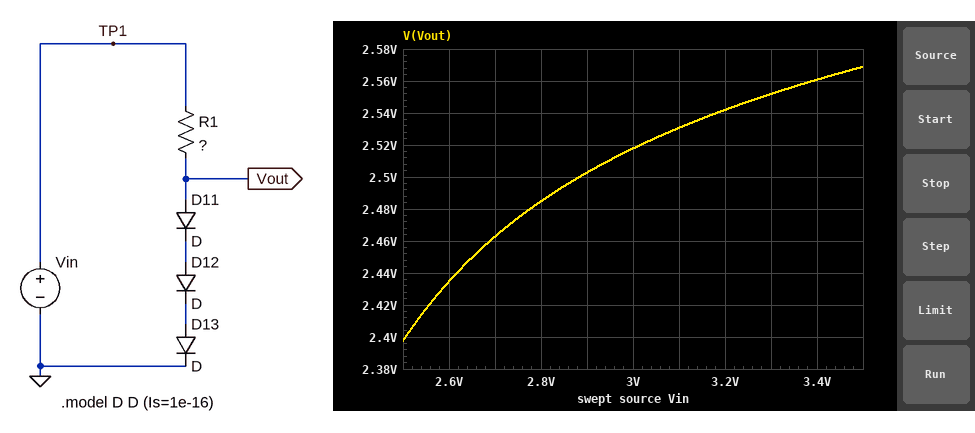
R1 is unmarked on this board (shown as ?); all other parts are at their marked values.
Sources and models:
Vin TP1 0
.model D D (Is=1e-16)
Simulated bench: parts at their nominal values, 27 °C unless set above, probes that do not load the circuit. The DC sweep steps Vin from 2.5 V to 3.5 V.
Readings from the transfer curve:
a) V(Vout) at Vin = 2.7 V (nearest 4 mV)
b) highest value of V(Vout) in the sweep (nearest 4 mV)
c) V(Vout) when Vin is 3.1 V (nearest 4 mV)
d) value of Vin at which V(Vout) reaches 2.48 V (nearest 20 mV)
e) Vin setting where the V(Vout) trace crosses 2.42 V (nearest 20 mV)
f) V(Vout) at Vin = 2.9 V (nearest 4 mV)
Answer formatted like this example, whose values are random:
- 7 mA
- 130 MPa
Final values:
- 2.464 V
- 2.568 V
- 2.532 V
- 2.78 V
- 2.56 V
- 2.504 V
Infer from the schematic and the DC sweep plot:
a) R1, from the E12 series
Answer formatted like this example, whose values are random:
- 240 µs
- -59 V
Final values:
- 39 Ω
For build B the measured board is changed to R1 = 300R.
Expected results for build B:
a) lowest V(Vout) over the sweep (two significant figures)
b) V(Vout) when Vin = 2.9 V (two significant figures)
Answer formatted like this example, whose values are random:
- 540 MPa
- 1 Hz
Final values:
- 2.3 V
- 2.4 V
